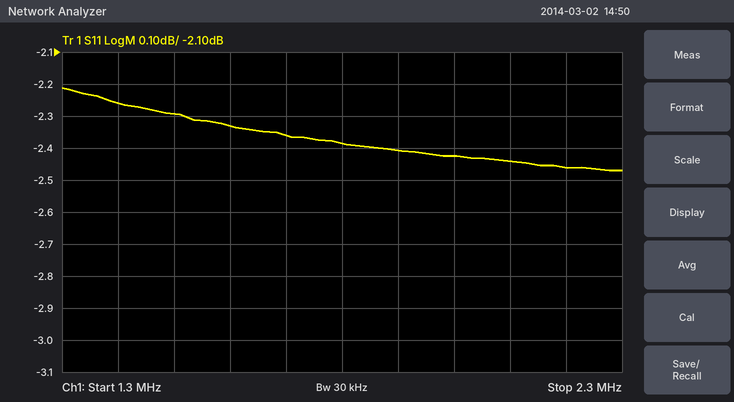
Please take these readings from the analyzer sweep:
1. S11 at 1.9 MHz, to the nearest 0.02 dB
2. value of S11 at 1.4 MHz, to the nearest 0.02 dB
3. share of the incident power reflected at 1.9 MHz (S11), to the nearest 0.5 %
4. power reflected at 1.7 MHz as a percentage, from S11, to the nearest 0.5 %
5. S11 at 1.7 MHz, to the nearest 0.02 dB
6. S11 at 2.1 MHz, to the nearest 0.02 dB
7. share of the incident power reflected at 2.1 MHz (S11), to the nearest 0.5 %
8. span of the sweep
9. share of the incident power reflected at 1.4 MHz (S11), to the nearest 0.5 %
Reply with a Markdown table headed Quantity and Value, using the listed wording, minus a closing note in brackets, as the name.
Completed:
| Quantity | Value |
|---|---|
| S11 at 1.9 MHz, to the nearest 0.02 dB | -2.40 dB |
| value of S11 at 1.4 MHz, to the nearest 0.02 dB | -2.26 dB |
| share of the incident power reflected at 1.9 MHz (S11), to the nearest 0.5 % | 57.5 % |
| power reflected at 1.7 MHz as a percentage, from S11, to the nearest 0.5 % | 58.0 % |
| S11 at 1.7 MHz, to the nearest 0.02 dB | -2.36 dB |
| S11 at 2.1 MHz, to the nearest 0.02 dB | -2.44 dB |
| share of the incident power reflected at 2.1 MHz (S11), to the nearest 0.5 % | 57.0 % |
| span of the sweep | 1 MHz |
| share of the incident power reflected at 1.4 MHz (S11), to the nearest 0.5 % | 59.5 % |
